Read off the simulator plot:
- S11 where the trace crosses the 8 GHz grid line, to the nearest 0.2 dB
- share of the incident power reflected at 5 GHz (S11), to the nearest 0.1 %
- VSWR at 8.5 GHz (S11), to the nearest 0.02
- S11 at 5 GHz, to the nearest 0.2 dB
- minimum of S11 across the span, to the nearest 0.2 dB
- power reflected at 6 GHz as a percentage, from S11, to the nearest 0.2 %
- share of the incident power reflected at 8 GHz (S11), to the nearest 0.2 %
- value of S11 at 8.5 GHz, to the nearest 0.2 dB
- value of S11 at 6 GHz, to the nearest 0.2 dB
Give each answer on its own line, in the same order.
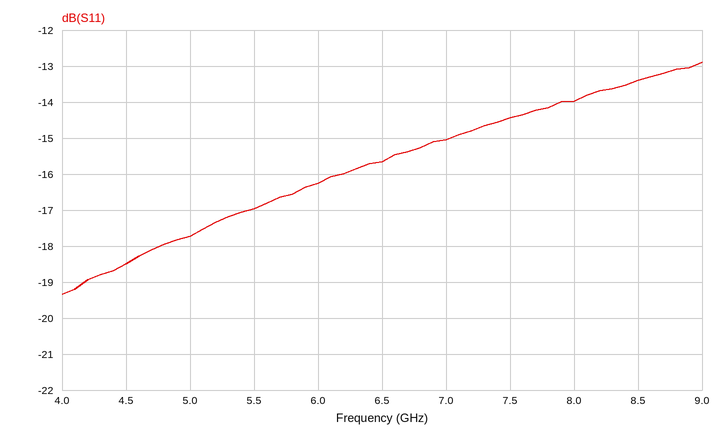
-14.0 dB
1.7 %
1.54
-17.8 dB
-19.4 dB
2.4 %
4.0 %
-13.4 dB
-16.2 dB
